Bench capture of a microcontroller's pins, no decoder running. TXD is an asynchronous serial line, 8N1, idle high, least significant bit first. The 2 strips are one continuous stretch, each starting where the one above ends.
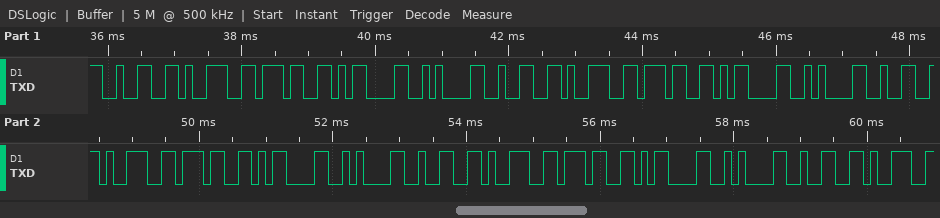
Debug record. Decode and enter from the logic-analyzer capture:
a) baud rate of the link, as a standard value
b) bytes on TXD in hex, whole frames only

9600 baud
32 39 37 0D 0A 32 39 37 0D 0A 32 39 37 0D 0A 32 39 37 0D 0A 32 39
